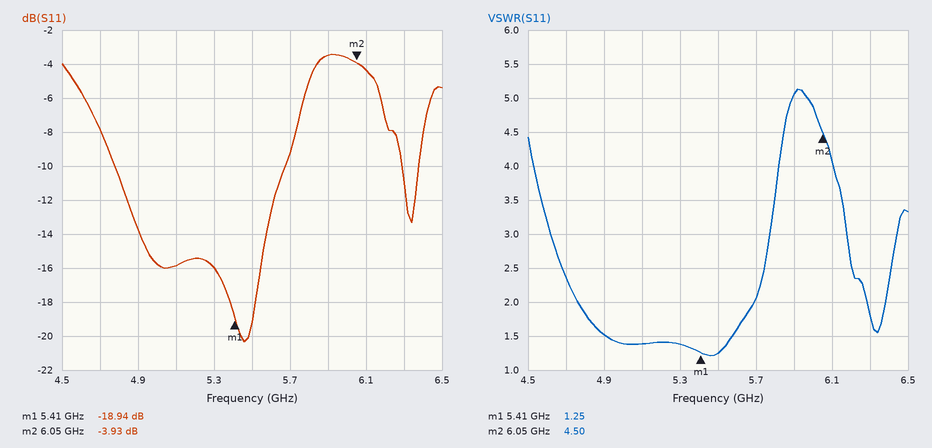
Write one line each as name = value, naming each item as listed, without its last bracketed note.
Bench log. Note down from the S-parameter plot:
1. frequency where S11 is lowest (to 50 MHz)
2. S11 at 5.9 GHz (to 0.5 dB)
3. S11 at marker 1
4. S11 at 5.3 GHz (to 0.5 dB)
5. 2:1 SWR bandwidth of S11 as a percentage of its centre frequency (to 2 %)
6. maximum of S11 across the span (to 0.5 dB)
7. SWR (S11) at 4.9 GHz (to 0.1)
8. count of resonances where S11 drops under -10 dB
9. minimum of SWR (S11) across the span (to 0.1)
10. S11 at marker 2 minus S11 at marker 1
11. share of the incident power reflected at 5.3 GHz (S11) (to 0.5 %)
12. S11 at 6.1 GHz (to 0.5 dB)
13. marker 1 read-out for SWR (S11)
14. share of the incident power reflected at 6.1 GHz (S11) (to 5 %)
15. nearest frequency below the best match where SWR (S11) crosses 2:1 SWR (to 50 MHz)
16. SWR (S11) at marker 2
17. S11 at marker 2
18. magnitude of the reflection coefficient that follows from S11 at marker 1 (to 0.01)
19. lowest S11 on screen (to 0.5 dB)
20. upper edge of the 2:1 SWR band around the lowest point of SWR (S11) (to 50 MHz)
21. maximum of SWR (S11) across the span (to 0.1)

frequency where S11 is lowest = 5.45 GHz
S11 at 5.9 GHz = -3.5 dB
S11 at marker 1 = -18.94 dB
S11 at 5.3 GHz = -16.0 dB
2:1 SWR bandwidth of S11 as a percentage of its centre frequency = 18 %
maximum of S11 across the span = -3.5 dB
SWR (S11) at 4.9 GHz = 1.5
count of resonances where S11 drops under -10 dB = 2
minimum of SWR (S11) across the span = 1.2
S11 at marker 2 minus S11 at marker 1 = 15.01 dB
share of the incident power reflected at 5.3 GHz (S11) = 2.5 %
S11 at 6.1 GHz = -4.5 dB
marker 1 read-out for SWR = 1.25
share of the incident power reflected at 6.1 GHz (S11) = 35 %
nearest frequency below the best match where SWR (S11) crosses 2:1 SWR = 4.75 GHz
SWR (S11) at marker 2 = 4.50
S11 at marker 2 = -3.93 dB
magnitude of the reflection coefficient that follows from S11 at marker 1 = 0.11
lowest S11 on screen = -20.5 dB
upper edge of the 2:1 SWR band around the lowest point of SWR (S11) = 5.70 GHz
maximum of SWR (S11) across the span = 5.1
